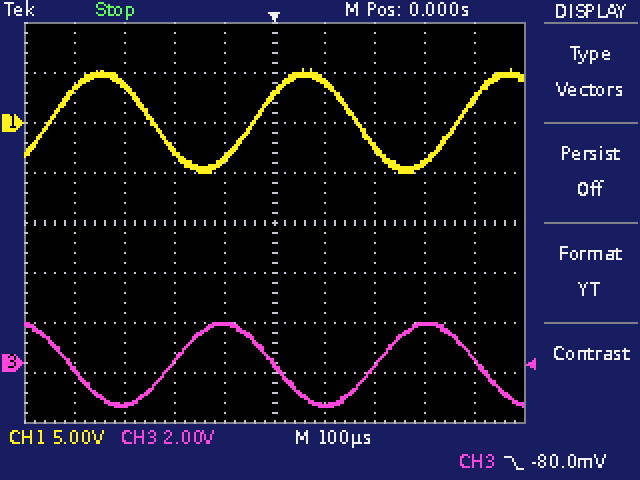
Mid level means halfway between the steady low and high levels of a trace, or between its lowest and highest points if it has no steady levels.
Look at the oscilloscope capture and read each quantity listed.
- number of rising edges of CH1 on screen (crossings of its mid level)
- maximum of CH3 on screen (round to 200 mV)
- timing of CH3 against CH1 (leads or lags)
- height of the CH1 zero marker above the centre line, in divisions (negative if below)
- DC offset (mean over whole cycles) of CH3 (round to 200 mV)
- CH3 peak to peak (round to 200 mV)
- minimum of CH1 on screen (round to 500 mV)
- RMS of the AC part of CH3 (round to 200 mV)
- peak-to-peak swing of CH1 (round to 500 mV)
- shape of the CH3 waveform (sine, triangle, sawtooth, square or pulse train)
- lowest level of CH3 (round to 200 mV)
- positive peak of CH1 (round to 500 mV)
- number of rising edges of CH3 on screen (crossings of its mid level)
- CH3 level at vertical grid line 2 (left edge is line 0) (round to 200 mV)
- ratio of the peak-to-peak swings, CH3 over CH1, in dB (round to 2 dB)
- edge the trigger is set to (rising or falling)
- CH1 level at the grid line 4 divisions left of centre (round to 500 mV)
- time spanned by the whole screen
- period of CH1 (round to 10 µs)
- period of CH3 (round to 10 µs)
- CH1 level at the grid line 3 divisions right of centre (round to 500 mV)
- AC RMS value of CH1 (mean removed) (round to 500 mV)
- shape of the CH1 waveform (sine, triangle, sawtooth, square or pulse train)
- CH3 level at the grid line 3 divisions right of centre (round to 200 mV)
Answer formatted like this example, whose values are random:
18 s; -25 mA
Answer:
3; 1.6 V; leads; +2.0 div; 0.0 V; 3.4 V; -5.0 V; 1.2 V; 10.5 V; sine; -1.8 V; 5.5 V; 2; -1.6 V; -10 dB; falling; 3.5 V; 1 ms; 410 µs; 410 µs; -4.0 V; 3.5 V; sine; 1.6 V
